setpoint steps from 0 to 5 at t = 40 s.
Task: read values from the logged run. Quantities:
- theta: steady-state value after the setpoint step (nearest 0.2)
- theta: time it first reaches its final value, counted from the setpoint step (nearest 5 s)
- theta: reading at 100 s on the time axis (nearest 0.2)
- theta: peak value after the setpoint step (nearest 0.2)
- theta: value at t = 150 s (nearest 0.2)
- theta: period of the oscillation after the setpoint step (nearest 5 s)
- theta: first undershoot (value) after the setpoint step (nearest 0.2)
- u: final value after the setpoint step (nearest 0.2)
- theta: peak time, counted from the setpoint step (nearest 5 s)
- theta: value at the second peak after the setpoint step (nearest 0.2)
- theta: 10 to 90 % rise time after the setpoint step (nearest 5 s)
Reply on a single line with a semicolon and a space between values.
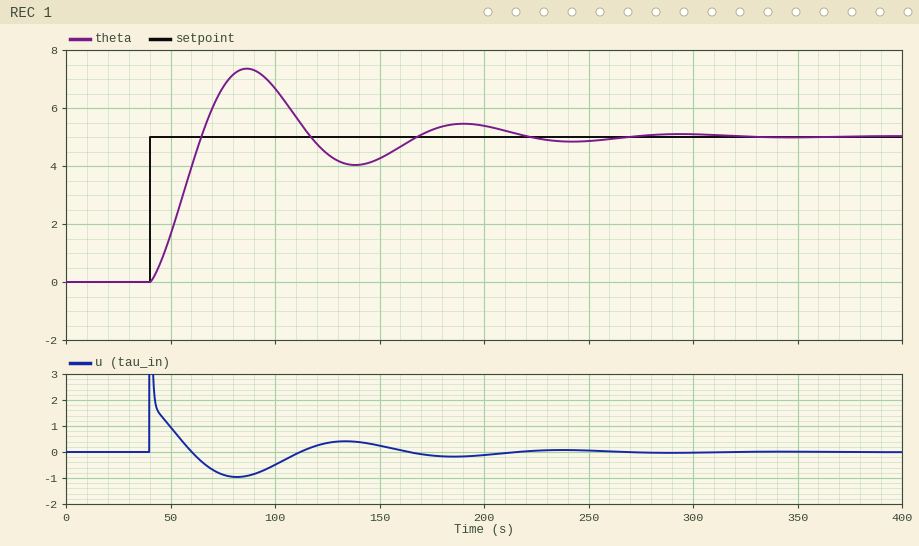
5.0; 25 s; 6.6; 7.4; 4.2; 105 s; 4.0; 0.0; 45 s; 5.4; 20 s
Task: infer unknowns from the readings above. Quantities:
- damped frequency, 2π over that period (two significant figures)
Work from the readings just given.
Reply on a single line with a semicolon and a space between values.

0.060 rad/s
